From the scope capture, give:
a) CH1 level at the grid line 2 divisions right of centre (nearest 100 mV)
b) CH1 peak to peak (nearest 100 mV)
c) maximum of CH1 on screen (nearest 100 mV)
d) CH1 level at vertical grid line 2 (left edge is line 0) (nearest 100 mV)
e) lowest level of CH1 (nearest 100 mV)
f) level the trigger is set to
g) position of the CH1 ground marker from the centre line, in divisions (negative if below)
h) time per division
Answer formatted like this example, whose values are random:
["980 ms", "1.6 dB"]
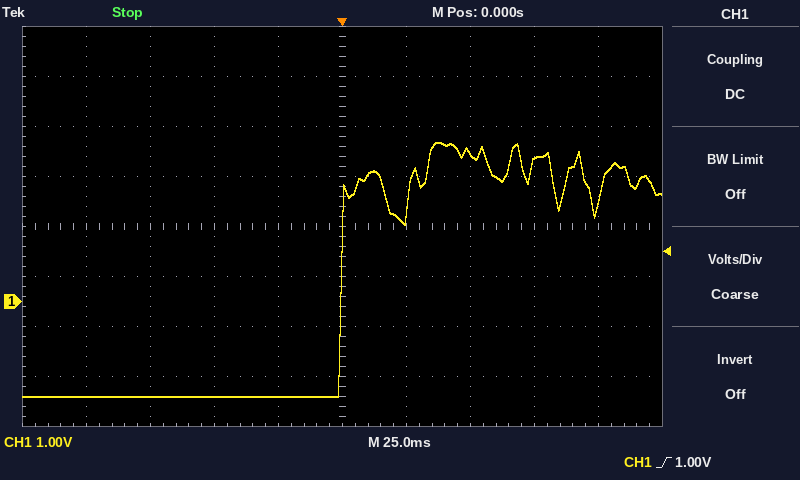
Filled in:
["3.0 V", "5.1 V", "3.2 V", "-1.9 V", "-1.9 V", "1.00 V", "-1.5 div", "25 ms"]
